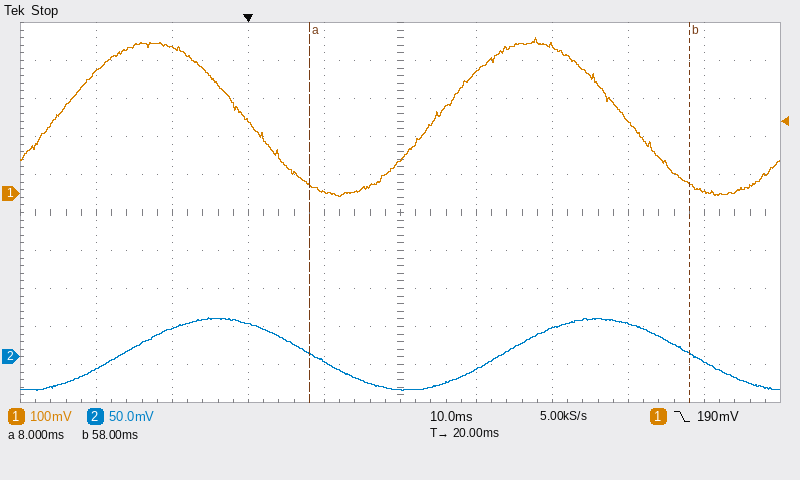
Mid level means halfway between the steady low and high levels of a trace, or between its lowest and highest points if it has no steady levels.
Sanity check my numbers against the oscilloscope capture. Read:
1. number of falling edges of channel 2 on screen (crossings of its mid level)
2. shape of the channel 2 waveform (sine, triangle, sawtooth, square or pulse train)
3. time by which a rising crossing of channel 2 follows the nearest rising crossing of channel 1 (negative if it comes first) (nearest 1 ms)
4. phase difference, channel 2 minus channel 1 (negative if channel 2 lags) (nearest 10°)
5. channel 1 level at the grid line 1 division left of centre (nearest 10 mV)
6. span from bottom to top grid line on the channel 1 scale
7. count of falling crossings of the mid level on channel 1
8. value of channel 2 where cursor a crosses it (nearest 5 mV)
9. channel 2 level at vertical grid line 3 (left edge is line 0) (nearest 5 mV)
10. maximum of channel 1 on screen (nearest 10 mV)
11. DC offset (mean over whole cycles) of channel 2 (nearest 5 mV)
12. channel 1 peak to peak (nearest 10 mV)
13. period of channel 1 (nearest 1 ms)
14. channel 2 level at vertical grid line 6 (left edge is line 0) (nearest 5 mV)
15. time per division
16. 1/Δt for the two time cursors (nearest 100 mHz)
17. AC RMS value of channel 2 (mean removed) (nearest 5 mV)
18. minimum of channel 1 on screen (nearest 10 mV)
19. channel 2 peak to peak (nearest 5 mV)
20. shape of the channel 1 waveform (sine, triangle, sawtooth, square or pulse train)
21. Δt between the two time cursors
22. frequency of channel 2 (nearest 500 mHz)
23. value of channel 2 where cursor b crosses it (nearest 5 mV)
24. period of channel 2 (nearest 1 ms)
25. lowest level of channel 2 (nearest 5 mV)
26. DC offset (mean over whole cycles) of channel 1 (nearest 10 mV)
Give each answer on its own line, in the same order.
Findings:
2
sine
+9 ms
-60°
0 mV
1 V
2
5 mV
45 mV
410 mV
5 mV
420 mV
50 ms
-15 mV
10 ms
20.0 Hz
35 mV
-10 mV
95 mV
sine
50 ms
20.0 Hz
5 mV
50 ms
-45 mV
200 mV
